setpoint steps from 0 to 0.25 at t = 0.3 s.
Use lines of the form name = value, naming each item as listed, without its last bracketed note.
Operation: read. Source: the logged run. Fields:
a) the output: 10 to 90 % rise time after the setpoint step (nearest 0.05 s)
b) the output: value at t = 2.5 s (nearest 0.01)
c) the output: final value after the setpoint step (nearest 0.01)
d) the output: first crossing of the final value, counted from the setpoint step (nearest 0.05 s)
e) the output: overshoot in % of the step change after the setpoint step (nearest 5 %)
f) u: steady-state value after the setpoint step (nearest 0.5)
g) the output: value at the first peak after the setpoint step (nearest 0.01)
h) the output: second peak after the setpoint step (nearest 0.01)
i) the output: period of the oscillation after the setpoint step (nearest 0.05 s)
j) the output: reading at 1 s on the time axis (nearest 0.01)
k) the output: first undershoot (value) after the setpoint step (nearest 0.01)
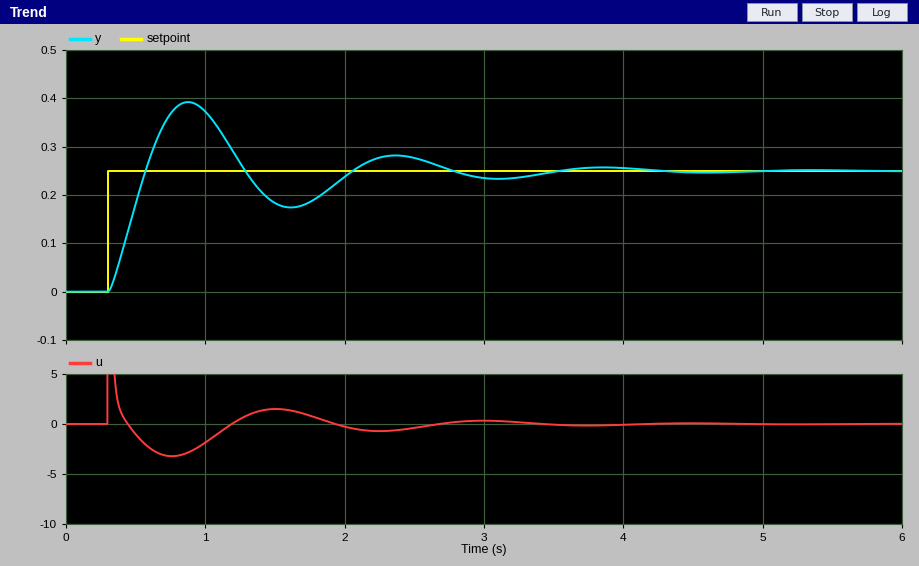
the output: 10 to 90 % rise time after the setpoint step = 0.20 s
the output: value at t = 2.5 s = 0.28
the output: final value after the setpoint step = 0.25
the output: first crossing of the final value, counted from the setpoint step = 0.25 s
the output: overshoot in % of the step change after the setpoint step = 55 %
u: steady-state value after the setpoint step = 0.0
the output: value at the first peak after the setpoint step = 0.39
the output: second peak after the setpoint step = 0.28
the output: period of the oscillation after the setpoint step = 1.50 s
the output: reading at 1 s on the time axis = 0.37
the output: first undershoot (value) after the setpoint step = 0.17
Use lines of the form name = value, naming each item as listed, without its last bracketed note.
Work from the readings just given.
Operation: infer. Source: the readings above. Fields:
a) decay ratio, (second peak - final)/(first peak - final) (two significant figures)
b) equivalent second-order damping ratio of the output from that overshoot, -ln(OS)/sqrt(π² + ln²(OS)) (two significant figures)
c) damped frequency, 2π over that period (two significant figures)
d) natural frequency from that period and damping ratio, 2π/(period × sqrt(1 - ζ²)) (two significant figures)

decay ratio, (second peak - final)/(first peak - final) = 0.21
equivalent second-order damping ratio of the output from that overshoot, -ln(OS)/sqrt(π² + ln²(OS)) = 0.19
damped frequency, 2π over that period = 4.2 rad/s
natural frequency from that period and damping ratio, 2π/(period × sqrt(1 - ζ²)) = 4.3 rad/s
